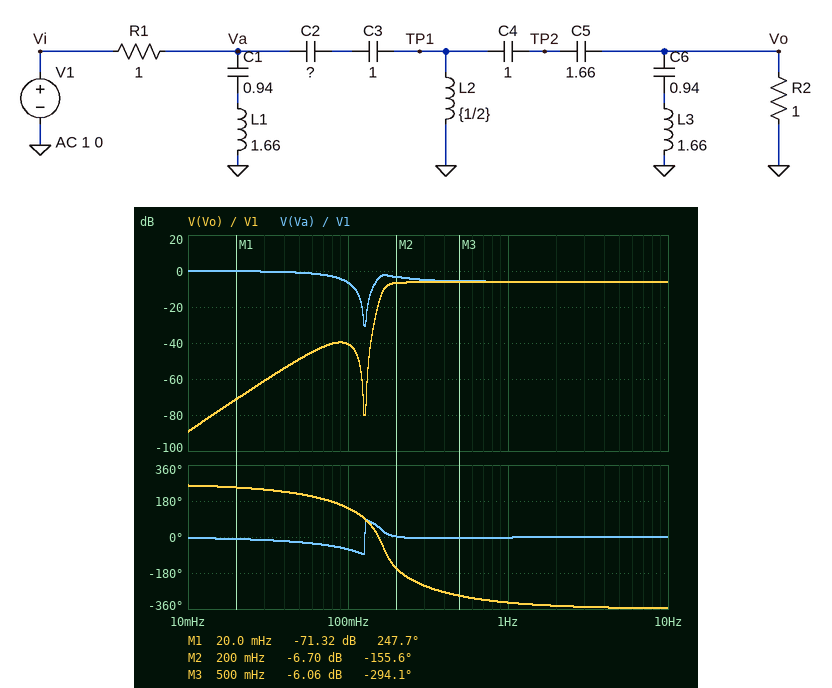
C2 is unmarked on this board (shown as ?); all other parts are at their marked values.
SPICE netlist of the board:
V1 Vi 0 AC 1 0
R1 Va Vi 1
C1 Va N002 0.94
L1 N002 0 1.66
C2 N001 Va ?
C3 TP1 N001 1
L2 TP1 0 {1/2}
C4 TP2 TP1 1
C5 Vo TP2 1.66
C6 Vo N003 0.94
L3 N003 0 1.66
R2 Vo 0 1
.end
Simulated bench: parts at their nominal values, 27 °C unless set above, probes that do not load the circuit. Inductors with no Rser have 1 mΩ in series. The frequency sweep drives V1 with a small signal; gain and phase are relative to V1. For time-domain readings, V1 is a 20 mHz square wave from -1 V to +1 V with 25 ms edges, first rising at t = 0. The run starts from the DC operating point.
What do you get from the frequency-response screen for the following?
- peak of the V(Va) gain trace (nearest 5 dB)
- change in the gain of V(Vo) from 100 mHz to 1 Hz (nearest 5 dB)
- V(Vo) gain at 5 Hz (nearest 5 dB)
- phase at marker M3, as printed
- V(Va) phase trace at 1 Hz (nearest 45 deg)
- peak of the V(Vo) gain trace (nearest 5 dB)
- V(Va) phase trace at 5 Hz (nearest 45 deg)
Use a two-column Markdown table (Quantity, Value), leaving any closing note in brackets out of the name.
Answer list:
| Quantity | Value |
|---|---|
| peak of the V(Va) gain trace | 0 dB |
| change in the gain of V(Vo) from 100 mHz to 1 Hz | 35 dB |
| V(Vo) gain at 5 Hz | -5 dB |
| phase at marker M3, as printed | -294.1 deg |
| V(Va) phase trace at 1 Hz | 0 deg |
| peak of the V(Vo) gain trace | -5 dB |
| V(Va) phase trace at 5 Hz | 0 deg |
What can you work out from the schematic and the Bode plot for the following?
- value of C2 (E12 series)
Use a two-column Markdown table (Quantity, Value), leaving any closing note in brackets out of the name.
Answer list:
| Quantity | Value |
|---|---|
| value of C2 | 820 mF |
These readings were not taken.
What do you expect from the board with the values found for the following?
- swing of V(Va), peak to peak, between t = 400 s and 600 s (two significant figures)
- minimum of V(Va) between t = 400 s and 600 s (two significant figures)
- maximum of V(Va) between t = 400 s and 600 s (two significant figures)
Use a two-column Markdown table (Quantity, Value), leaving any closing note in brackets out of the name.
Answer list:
| Quantity | Value |
|---|---|
| swing of V(Va), peak to peak, between t = 400 s and 600 s | 2.5 V |
| minimum of V(Va) between t = 400 s and 600 s | -1.2 V |
| maximum of V(Va) between t = 400 s and 600 s | 1.2 V |
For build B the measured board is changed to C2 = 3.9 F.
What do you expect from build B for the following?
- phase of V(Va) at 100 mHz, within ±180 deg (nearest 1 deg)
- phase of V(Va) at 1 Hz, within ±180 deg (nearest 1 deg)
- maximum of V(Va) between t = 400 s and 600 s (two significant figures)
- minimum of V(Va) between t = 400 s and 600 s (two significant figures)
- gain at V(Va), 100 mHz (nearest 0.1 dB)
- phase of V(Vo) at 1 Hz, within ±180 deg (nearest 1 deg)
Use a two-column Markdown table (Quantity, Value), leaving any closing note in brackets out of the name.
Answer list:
| Quantity | Value |
|---|---|
| phase of V(Va) at 100 mHz, within ±180 deg | -65 deg |
| phase of V(Va) at 1 Hz, within ±180 deg | 2 deg |
| maximum of V(Va) between t = 400 s and 600 s | 1.1 V |
| minimum of V(Va) between t = 400 s and 600 s | -1.1 V |
| gain at V(Va), 100 mHz | -7.5 dB |
| phase of V(Vo) at 1 Hz, within ±180 deg | 28 deg |
